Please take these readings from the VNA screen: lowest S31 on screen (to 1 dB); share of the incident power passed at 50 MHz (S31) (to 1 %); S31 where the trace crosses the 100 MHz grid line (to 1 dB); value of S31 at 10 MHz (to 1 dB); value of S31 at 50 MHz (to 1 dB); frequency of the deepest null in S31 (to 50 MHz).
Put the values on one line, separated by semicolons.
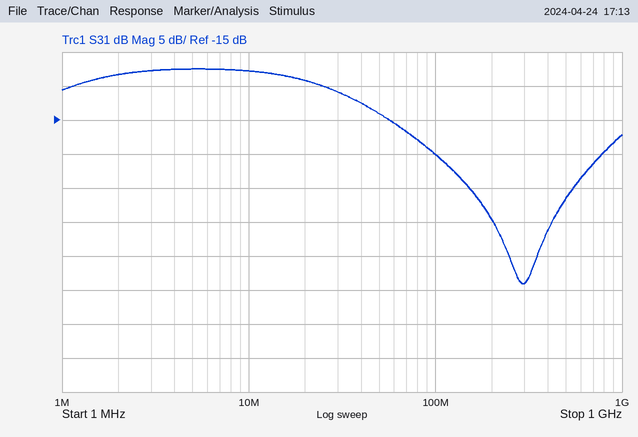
-39 dB; 4 %; -20 dB; -8 dB; -14 dB; 300 MHz
